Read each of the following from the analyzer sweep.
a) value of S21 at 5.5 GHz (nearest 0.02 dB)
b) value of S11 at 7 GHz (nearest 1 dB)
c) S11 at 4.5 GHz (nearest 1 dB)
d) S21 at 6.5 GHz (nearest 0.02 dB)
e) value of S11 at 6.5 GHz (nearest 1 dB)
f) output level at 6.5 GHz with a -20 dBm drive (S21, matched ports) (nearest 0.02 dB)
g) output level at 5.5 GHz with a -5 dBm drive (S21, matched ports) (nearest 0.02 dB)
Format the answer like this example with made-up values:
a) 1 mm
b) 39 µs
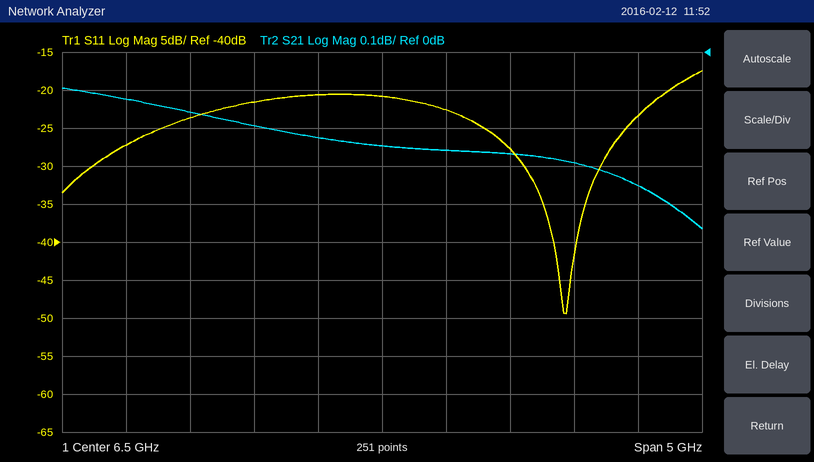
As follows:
a) -0.20 dB
b) -23 dB
c) -27 dB
d) -0.24 dB
e) -21 dB
f) -20.24 dBm
g) -5.20 dBm
